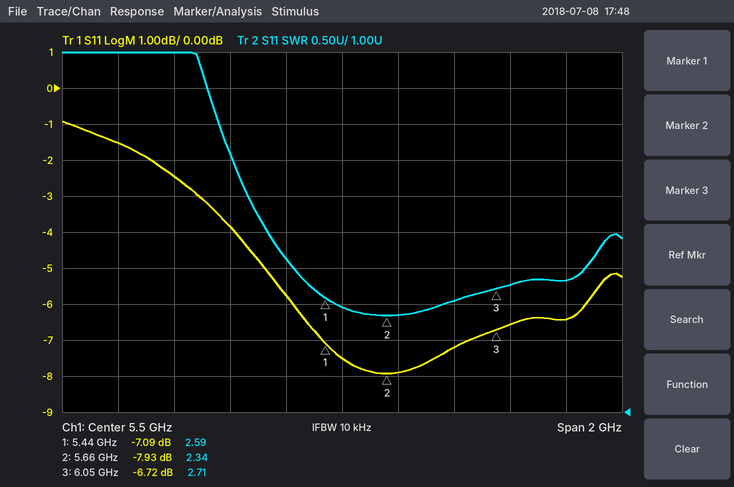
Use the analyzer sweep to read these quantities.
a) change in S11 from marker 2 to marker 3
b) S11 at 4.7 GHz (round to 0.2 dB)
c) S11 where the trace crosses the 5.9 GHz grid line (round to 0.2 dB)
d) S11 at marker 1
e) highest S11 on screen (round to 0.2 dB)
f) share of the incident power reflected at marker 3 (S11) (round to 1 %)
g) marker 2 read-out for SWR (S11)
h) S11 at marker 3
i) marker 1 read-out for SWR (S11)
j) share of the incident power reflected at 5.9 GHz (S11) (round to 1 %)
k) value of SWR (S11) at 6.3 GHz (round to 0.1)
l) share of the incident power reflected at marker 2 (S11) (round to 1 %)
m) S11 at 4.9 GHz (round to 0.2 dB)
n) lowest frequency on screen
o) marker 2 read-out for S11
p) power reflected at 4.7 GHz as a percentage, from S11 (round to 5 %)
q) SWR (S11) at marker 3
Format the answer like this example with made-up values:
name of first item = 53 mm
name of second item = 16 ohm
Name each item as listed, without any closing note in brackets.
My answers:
change in S11 from marker 2 to marker 3 = 1.21 dB
S11 at 4.7 GHz = -1.6 dB
S11 where the trace crosses the 5.9 GHz grid line = -7.2 dB
S11 at marker 1 = -7.09 dB
highest S11 on screen = -1.0 dB
share of the incident power reflected at marker 3 (S11) = 21 %
marker 2 read-out for SWR = 2.34
S11 at marker 3 = -6.72 dB
marker 1 read-out for SWR = 2.59
share of the incident power reflected at 5.9 GHz (S11) = 19 %
value of SWR (S11) at 6.3 GHz = 2.8
share of the incident power reflected at marker 2 (S11) = 16 %
S11 at 4.9 GHz = -2.4 dB
lowest frequency on screen = 4.5 GHz
marker 2 read-out for S11 = -7.93 dB
power reflected at 4.7 GHz as a percentage, from S11 = 70 %
SWR (S11) at marker 3 = 2.71
